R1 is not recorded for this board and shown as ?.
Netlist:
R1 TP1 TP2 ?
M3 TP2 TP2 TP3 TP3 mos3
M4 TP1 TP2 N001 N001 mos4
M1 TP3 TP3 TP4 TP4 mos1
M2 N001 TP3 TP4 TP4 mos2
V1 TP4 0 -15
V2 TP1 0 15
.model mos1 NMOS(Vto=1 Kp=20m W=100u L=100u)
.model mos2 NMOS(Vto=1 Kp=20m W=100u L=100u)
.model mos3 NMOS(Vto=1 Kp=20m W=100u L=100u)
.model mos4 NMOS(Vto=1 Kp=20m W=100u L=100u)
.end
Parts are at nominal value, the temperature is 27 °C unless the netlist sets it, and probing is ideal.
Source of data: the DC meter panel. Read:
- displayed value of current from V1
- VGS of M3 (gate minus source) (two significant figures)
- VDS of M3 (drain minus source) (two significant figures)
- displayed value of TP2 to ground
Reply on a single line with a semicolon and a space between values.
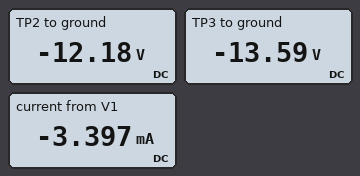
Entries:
-3.397 mA; 1.4 V; 1.4 V; -12.18 V
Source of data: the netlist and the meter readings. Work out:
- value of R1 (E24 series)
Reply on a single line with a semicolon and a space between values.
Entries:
16 kΩ
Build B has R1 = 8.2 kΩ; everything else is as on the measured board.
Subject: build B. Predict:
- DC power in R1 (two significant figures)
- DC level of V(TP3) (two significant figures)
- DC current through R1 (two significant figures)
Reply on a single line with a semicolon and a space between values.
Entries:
88 mW; -13 V; 3.3 mA
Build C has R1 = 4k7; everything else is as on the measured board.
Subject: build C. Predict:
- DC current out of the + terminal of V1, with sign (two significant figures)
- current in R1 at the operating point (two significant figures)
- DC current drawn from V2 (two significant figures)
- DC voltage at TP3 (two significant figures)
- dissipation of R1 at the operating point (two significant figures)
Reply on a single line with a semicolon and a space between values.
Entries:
-11 mA; 5.6 mA; 11 mA; -13 V; 150 mW
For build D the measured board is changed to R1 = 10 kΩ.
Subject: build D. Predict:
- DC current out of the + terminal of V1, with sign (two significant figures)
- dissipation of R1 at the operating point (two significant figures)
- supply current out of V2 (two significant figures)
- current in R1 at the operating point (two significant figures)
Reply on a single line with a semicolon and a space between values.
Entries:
-5.4 mA; 73 mW; 5.4 mA; 2.7 mA
